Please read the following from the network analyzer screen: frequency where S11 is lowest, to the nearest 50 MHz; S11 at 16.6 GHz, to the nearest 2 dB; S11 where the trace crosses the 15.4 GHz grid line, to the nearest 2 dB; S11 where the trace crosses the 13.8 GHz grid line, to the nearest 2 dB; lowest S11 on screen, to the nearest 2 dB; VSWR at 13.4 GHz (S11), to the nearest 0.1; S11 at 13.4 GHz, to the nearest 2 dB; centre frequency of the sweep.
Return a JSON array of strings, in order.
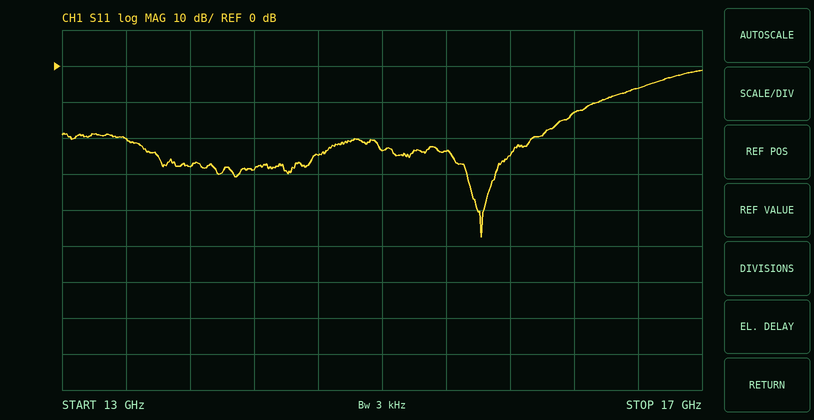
["15.60 GHz", "-6 dB", "-24 dB", "-28 dB", "-48 dB", "1.2", "-20 dB", "15 GHz"]
